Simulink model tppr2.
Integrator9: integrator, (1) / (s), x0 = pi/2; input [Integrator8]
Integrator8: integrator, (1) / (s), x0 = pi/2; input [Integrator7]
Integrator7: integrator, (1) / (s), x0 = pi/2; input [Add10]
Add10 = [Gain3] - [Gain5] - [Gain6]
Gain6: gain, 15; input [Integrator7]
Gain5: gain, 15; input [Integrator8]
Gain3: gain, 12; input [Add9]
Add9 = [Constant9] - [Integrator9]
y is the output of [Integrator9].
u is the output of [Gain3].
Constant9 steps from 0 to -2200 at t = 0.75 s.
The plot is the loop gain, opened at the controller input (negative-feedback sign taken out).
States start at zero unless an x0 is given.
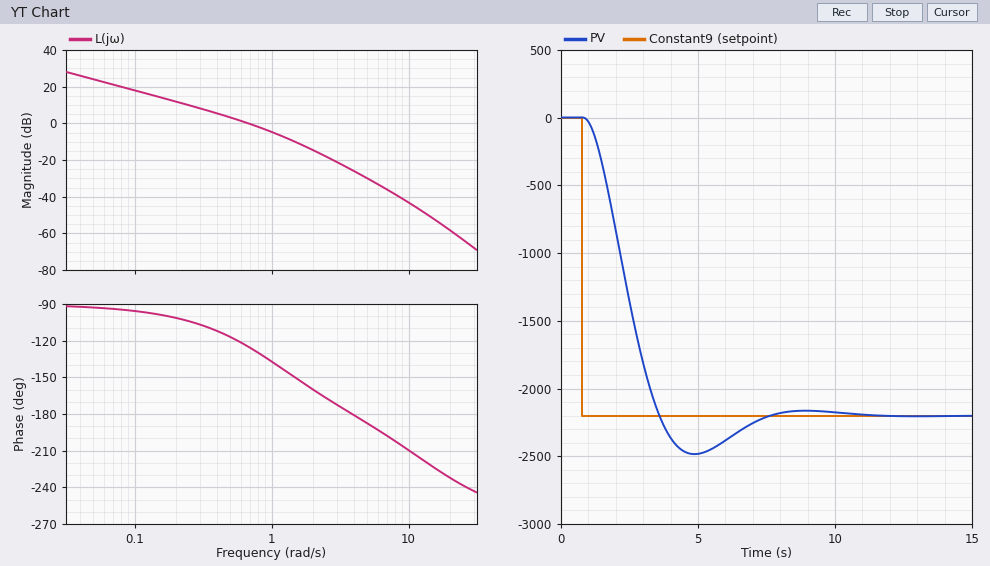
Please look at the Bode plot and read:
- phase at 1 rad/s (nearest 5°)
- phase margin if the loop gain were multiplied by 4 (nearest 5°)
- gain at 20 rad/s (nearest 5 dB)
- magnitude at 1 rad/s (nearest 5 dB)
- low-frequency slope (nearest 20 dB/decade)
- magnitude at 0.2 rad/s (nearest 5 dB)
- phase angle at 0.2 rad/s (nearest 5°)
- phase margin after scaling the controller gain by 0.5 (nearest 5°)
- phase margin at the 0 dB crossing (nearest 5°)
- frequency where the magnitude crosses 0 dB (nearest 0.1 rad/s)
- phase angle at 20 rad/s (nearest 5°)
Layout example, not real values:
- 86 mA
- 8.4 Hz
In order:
- -135°
- 25°
- -60 dB
- -5 dB
- -20 dB/decade
- 10 dB
- -100°
- 70°
- 55°
- 0.7 rad/s
- -230°
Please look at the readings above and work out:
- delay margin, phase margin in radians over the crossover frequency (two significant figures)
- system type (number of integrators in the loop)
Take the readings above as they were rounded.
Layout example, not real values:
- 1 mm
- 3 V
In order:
- 1.4 s
- 1
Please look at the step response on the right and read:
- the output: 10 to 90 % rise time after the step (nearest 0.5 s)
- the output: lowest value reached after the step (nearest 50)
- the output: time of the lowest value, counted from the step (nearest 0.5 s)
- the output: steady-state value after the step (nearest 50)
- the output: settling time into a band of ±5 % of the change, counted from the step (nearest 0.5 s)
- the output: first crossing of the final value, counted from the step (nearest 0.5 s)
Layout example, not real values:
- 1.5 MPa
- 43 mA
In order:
- 2.0 s
- -2500
- 4.0 s
- -2200
- 6.0 s
- 3.0 s
